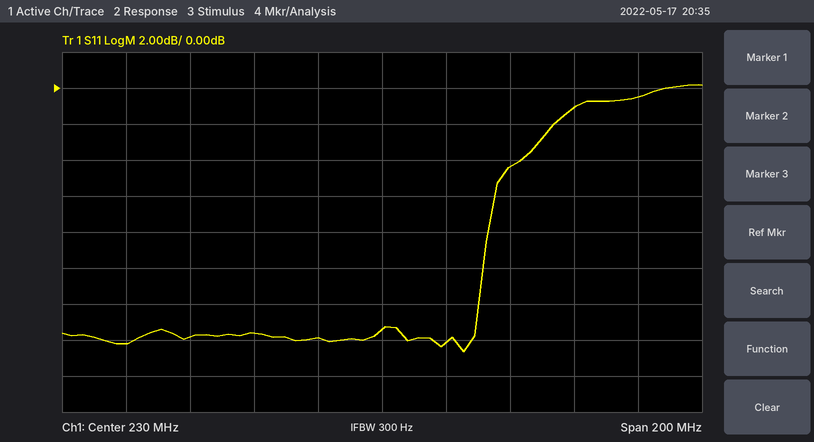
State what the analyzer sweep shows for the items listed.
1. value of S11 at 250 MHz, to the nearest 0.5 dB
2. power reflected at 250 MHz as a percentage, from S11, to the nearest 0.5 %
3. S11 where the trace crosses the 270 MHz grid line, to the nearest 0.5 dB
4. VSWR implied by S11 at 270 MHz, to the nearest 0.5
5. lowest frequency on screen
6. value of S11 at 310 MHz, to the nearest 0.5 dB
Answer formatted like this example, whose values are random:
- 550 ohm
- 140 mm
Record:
- -14.0 dB
- 4.0 %
- -4.5 dB
- 4.0
- 130 MHz
- -0.5 dB
